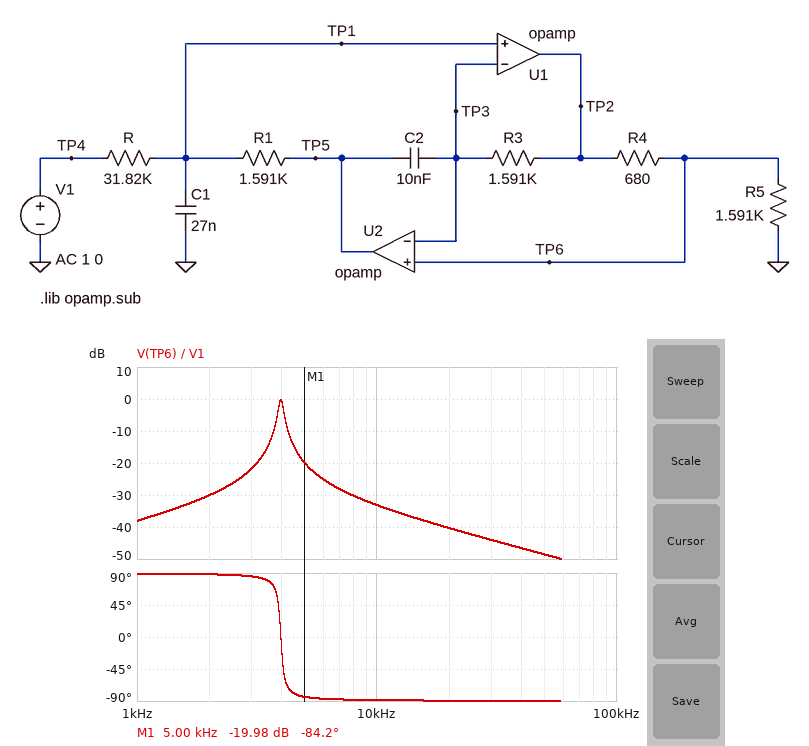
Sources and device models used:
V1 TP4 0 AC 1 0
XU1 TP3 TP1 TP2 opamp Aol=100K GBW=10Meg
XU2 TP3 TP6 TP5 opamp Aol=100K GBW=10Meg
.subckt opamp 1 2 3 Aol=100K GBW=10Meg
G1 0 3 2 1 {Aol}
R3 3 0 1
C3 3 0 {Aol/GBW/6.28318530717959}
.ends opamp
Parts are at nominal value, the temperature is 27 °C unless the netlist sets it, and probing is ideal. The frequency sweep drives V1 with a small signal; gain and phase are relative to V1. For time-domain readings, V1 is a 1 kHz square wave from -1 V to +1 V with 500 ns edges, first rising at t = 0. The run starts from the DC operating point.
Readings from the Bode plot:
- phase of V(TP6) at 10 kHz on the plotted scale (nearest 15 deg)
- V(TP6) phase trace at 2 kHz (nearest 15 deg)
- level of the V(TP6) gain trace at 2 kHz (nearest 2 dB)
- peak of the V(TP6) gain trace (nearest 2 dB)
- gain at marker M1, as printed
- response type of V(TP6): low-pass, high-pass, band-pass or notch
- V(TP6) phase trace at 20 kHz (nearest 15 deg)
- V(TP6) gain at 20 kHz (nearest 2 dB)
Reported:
-90 deg
90 deg
-30 dB
0 dB
-19.98 dB
band-pass
-90 deg
-40 dB
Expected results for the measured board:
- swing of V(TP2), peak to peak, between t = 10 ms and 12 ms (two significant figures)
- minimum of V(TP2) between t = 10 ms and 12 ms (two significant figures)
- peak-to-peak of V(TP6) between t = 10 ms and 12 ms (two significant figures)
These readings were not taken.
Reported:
150 mV
-74 mV
100 mV
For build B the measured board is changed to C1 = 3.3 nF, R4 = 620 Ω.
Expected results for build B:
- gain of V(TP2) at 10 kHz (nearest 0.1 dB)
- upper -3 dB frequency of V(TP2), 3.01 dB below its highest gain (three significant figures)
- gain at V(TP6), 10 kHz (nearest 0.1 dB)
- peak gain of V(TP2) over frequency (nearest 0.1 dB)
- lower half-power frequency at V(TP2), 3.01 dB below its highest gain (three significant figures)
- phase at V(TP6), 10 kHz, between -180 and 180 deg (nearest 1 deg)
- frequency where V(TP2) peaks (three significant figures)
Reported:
-0.9 dB
11.6 kHz
-3.8 dB
2.7 dB
10.1 kHz
49 deg
10.8 kHz
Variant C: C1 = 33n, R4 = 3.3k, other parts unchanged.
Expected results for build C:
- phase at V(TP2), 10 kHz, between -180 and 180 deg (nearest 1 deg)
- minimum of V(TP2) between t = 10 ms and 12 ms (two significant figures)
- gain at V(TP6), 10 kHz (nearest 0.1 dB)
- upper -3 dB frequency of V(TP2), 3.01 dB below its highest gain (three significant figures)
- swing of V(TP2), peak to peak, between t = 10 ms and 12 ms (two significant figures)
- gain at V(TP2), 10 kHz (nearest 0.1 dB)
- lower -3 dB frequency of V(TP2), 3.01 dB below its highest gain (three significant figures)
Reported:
-88 deg
-65 mV
-27.9 dB
7.99 kHz
130 mV
-18.1 dB
7.84 kHz
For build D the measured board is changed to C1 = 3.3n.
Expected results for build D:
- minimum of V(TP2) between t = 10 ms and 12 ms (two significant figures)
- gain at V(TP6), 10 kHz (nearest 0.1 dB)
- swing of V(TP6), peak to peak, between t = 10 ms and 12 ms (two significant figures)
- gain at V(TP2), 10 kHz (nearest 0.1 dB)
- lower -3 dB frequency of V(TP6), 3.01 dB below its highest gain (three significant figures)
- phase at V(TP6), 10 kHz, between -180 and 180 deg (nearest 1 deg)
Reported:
-360 mV
-6.7 dB
510 mV
-3.6 dB
10.6 kHz
62 deg
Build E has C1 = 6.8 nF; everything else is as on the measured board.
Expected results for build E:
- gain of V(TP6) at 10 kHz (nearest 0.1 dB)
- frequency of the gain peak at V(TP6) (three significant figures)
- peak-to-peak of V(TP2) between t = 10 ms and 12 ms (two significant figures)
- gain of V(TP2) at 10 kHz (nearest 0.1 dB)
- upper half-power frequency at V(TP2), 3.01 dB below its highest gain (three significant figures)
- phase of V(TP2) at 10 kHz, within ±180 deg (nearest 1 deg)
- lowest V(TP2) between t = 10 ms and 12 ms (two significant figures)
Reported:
-14.3 dB
7.92 kHz
380 mV
-11.2 dB
8.30 kHz
-79 deg
-190 mV
